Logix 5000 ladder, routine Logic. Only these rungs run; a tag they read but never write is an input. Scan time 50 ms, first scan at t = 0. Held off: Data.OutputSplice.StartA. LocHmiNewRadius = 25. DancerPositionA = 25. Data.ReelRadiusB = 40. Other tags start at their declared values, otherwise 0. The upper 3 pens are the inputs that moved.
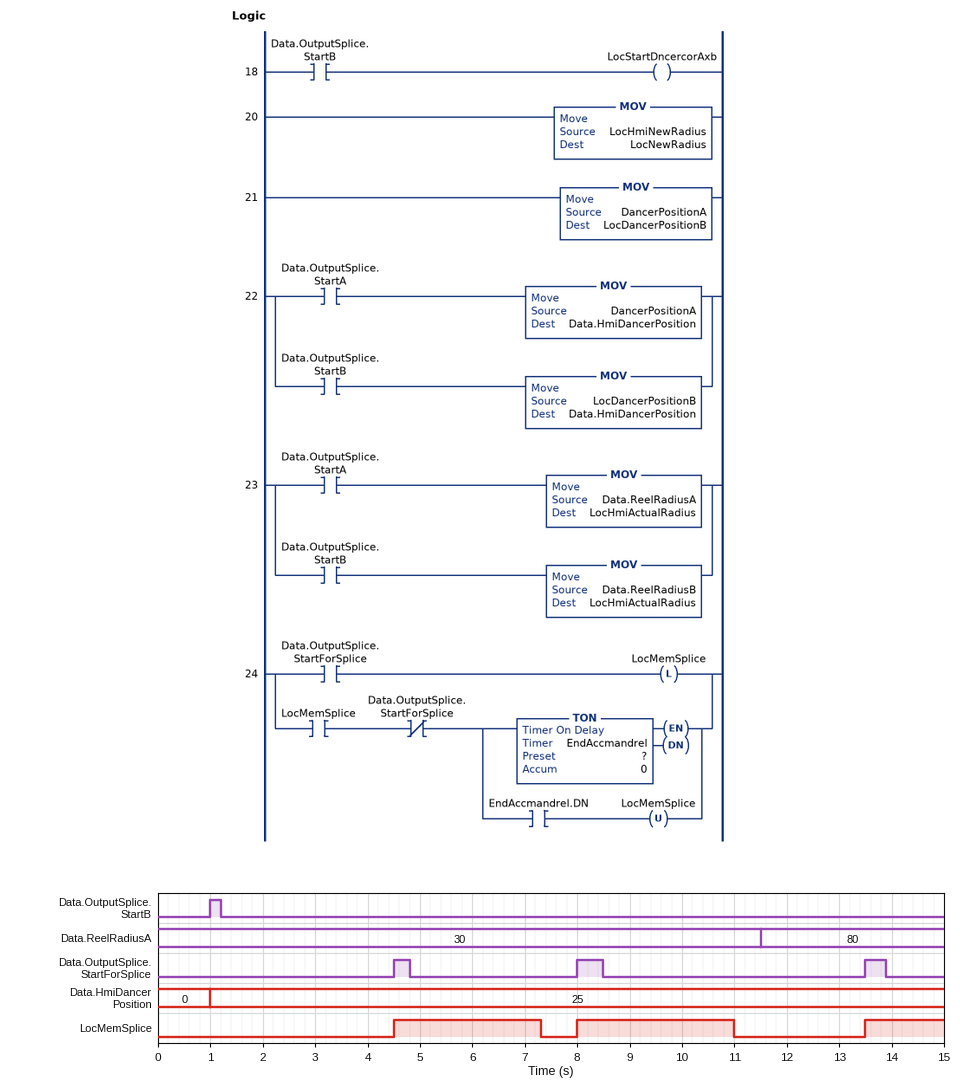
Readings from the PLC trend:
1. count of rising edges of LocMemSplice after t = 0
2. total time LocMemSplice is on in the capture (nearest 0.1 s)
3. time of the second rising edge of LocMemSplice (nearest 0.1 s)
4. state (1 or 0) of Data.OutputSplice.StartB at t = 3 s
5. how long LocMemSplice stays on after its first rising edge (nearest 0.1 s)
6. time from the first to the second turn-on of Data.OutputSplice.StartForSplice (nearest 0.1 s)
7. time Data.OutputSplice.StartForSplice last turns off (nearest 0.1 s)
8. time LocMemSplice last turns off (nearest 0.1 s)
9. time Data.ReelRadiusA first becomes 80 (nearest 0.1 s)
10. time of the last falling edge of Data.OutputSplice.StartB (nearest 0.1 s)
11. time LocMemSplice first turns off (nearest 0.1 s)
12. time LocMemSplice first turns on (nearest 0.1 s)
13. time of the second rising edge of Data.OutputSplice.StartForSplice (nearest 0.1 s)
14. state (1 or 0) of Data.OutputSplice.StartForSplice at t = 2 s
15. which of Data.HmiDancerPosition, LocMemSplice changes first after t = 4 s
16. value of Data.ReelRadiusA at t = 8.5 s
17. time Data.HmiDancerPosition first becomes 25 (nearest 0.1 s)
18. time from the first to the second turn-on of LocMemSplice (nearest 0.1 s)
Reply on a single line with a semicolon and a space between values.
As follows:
3; 7.3 s; 8.0 s; 0; 2.8 s; 3.5 s; 13.9 s; 11.0 s; 11.5 s; 1.2 s; 7.3 s; 4.5 s; 8.0 s; 0; LocMemSplice; 30; 1.0 s; 3.5 s
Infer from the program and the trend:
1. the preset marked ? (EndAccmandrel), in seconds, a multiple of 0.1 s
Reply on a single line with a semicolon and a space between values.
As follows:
2.5 s
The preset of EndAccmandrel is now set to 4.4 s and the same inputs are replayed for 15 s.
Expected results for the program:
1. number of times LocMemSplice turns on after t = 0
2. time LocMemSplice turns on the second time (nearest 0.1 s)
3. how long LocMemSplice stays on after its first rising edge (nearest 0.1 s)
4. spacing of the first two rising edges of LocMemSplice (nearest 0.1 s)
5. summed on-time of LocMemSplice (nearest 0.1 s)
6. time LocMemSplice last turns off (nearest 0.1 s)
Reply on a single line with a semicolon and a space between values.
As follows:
2; 13.5 s; 8.4 s; 9.0 s; 9.9 s; 12.9 s
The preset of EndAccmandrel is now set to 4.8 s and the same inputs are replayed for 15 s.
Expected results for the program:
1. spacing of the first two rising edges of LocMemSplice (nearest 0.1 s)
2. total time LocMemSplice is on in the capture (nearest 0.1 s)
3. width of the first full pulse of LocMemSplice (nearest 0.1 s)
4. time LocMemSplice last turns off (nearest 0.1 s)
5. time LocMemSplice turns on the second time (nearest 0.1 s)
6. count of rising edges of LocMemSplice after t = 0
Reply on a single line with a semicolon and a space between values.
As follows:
9.0 s; 10.3 s; 8.8 s; 13.3 s; 13.5 s; 2
